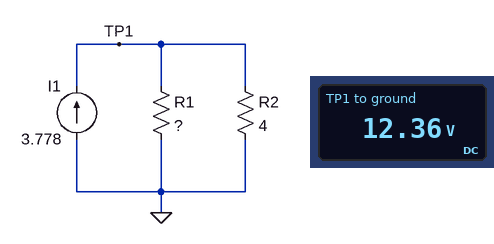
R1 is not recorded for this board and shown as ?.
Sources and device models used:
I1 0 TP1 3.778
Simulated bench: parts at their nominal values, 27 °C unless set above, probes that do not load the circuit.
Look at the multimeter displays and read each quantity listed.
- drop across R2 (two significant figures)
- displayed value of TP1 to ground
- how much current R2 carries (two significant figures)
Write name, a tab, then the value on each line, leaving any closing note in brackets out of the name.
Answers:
drop across R2	12 V
displayed value of TP1 to ground	12.36 V
how much current R2 carries	3.1 A
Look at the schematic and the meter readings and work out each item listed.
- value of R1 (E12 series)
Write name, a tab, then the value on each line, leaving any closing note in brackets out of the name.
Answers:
value of R1	18 Ω
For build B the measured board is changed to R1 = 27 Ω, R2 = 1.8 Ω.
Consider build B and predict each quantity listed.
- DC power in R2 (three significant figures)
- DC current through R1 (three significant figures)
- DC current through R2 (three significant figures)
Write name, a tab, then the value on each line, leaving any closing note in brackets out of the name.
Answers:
DC power in R2	22.6 W
DC current through R1	236 mA
DC current through R2	3.54 A
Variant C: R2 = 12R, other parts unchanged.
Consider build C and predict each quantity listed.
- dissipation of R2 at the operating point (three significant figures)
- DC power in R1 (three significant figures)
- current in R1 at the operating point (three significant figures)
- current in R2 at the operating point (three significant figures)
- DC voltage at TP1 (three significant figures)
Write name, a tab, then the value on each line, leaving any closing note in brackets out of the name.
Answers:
dissipation of R2 at the operating point	61.7 W
DC power in R1	41.1 W
current in R1 at the operating point	1.51 A
current in R2 at the operating point	2.27 A
DC voltage at TP1	27.2 V
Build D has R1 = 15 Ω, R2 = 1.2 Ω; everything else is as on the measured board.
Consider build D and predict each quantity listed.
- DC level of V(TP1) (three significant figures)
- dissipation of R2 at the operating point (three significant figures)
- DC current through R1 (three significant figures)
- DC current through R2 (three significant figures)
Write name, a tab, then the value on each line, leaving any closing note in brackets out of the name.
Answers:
DC level of V(TP1)	4.20 V
dissipation of R2 at the operating point	14.7 W
DC current through R1	280 mA
DC current through R2	3.50 A
